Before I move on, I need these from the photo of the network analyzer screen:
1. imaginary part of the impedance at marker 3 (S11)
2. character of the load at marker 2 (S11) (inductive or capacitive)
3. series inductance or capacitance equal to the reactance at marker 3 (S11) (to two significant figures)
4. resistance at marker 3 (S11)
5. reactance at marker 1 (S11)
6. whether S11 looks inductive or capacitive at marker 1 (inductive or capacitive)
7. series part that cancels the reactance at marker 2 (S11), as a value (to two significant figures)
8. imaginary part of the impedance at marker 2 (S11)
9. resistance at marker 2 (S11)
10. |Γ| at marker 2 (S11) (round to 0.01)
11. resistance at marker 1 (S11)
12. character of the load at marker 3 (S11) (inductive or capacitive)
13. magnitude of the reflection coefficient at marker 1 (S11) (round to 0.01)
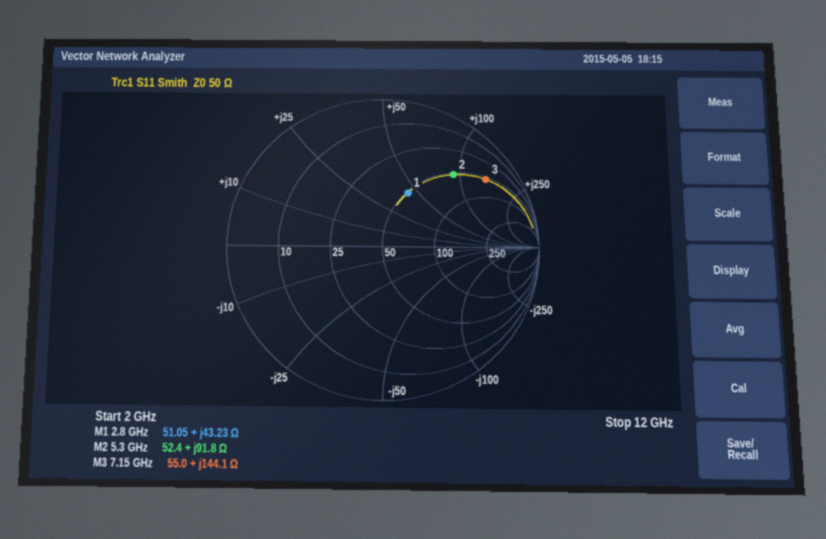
+144.1 Ω
inductive
3.2 nH
55.0 Ω
+43.23 Ω
inductive
330 fF
+91.8 Ω
52.4 Ω
0.67
51.05 Ω
inductive
0.39
